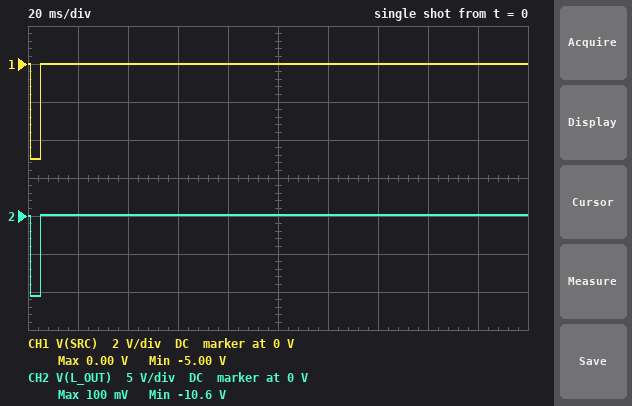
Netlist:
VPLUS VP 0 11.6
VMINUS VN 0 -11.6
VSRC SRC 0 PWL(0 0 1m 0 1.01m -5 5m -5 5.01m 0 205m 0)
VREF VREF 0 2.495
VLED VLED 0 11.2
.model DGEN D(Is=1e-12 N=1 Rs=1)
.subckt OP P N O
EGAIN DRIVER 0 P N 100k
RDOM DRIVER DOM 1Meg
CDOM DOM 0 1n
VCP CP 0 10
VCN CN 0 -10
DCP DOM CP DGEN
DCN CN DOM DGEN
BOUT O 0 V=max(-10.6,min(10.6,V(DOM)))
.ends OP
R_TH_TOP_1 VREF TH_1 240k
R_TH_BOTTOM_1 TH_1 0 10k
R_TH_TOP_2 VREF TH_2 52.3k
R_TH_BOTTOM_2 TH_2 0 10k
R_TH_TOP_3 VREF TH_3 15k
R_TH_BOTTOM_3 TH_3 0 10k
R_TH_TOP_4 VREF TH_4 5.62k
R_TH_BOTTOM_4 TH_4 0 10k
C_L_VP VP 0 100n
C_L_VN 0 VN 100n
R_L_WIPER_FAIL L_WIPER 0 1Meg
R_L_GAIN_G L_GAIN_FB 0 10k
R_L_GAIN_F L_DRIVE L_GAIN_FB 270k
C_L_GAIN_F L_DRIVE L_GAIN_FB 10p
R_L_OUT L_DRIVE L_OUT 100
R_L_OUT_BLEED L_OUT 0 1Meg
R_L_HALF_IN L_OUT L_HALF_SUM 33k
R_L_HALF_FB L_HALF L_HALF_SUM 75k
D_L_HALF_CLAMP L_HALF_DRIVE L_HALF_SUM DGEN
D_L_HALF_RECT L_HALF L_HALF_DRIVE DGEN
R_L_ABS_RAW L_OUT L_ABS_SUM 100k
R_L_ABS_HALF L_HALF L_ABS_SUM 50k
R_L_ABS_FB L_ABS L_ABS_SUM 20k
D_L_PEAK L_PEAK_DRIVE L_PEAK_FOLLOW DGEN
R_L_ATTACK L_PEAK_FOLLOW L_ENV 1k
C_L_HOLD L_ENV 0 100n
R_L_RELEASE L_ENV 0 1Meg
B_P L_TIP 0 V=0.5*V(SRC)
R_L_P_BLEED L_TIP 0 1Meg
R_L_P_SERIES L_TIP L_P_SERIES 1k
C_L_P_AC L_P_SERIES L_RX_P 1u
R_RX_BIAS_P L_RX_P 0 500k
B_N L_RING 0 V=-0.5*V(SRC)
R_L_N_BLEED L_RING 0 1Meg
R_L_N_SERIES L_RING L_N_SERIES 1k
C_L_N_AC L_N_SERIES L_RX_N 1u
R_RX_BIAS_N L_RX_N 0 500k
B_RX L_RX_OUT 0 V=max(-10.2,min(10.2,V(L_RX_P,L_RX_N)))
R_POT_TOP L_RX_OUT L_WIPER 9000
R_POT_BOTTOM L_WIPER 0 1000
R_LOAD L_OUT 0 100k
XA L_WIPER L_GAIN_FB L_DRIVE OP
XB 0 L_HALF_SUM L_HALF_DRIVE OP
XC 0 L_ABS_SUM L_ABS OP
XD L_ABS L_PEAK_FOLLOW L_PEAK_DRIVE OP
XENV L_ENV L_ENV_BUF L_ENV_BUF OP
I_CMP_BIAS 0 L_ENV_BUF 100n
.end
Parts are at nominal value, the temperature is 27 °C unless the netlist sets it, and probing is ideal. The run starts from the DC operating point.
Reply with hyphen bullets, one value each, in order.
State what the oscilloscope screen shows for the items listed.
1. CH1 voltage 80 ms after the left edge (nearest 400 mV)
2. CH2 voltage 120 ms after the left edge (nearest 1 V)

- 0 V
- 0 V
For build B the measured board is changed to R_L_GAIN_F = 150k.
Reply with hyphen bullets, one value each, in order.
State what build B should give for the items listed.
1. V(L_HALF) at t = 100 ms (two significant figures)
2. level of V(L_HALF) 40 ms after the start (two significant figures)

- -120 mV
- -130 mV
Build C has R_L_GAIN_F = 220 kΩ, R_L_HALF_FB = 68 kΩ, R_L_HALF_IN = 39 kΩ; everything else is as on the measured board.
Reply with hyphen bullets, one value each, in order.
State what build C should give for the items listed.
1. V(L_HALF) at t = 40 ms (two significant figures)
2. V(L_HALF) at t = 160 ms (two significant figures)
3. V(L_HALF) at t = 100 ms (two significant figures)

- -150 mV
- -120 mV
- -130 mV
